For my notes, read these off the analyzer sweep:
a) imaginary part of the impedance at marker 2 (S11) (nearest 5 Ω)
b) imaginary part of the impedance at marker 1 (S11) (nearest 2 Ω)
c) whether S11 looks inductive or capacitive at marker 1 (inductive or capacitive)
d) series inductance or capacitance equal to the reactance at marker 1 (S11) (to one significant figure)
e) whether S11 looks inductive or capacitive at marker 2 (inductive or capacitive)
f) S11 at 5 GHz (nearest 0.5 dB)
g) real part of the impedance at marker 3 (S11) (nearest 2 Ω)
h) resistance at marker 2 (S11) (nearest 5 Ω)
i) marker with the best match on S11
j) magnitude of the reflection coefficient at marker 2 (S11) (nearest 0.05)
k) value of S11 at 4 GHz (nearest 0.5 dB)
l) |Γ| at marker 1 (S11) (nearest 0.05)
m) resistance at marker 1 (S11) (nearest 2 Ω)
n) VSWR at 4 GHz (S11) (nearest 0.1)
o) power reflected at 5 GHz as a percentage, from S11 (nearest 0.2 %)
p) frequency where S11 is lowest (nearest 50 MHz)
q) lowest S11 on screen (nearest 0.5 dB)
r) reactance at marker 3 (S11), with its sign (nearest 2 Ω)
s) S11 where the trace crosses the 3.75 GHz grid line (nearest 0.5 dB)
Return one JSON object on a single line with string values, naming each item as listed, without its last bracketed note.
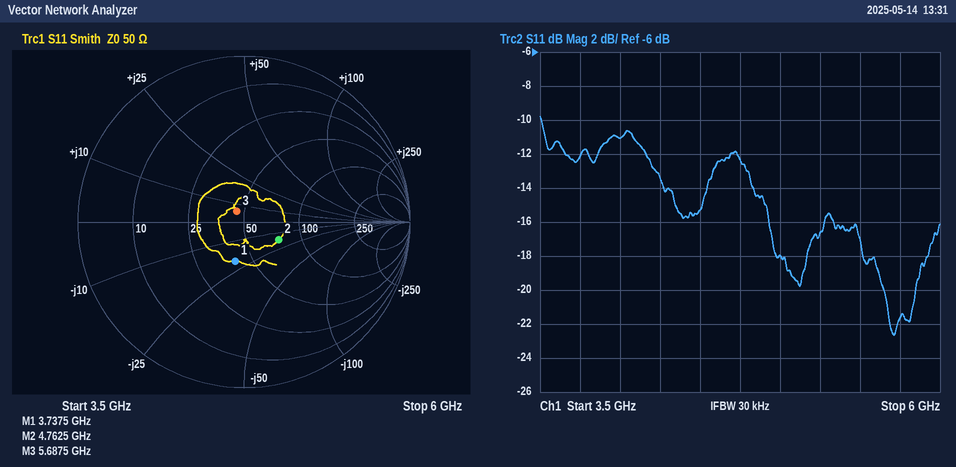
{"imaginary part of the impedance at marker 2 (S11)": "-15 Ω", "imaginary part of the impedance at marker 1 (S11)": "-20 Ω", "whether S11 looks inductive or capacitive at marker 1": "capacitive", "series inductance or capacitance equal to the reactance at marker 1 (S11)": "2 pF", "whether S11 looks inductive or capacitive at marker 2": "capacitive", "S11 at 5 GHz": "-18.0 dB", "real part of the impedance at marker 3 (S11)": "46 Ω", "resistance at marker 2 (S11)": "75 Ω", "marker with the best match on S11": "marker 3", "magnitude of the reflection coefficient at marker 2 (S11)": "0.25", "value of S11 at 4 GHz": "-11.0 dB", "|Γ| at marker 1 (S11)": "0.25", "resistance at marker 1 (S11)": "40 Ω", "VSWR at 4 GHz (S11)": "1.8", "power reflected at 5 GHz as a percentage, from S11": "1.6 %", "frequency where S11 is lowest": "5.70 GHz", "lowest S11 on screen": "-22.5 dB", "reactance at marker 3 (S11), with its sign": "+6 Ω", "S11 where the trace crosses the 3.75 GHz grid line": "-12.0 dB"}
